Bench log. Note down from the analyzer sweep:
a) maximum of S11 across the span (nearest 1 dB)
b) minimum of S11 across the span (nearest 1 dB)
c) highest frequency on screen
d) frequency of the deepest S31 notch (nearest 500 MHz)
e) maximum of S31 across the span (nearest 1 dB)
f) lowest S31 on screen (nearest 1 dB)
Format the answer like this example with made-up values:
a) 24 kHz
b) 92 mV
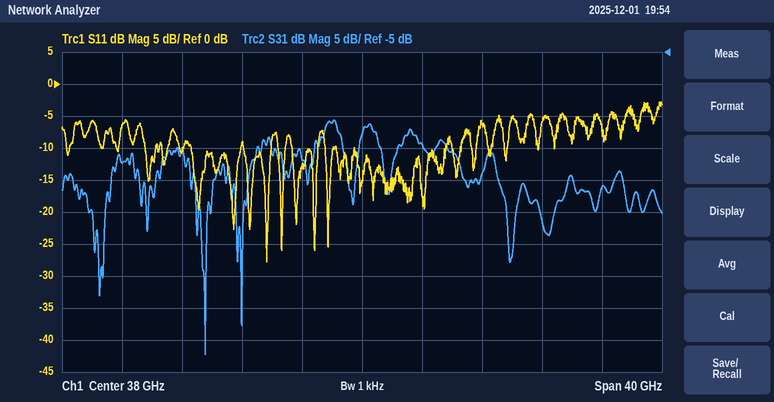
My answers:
a) -3 dB
b) -28 dB
c) 58 GHz
d) 27.5 GHz
e) -16 dB
f) -52 dB
